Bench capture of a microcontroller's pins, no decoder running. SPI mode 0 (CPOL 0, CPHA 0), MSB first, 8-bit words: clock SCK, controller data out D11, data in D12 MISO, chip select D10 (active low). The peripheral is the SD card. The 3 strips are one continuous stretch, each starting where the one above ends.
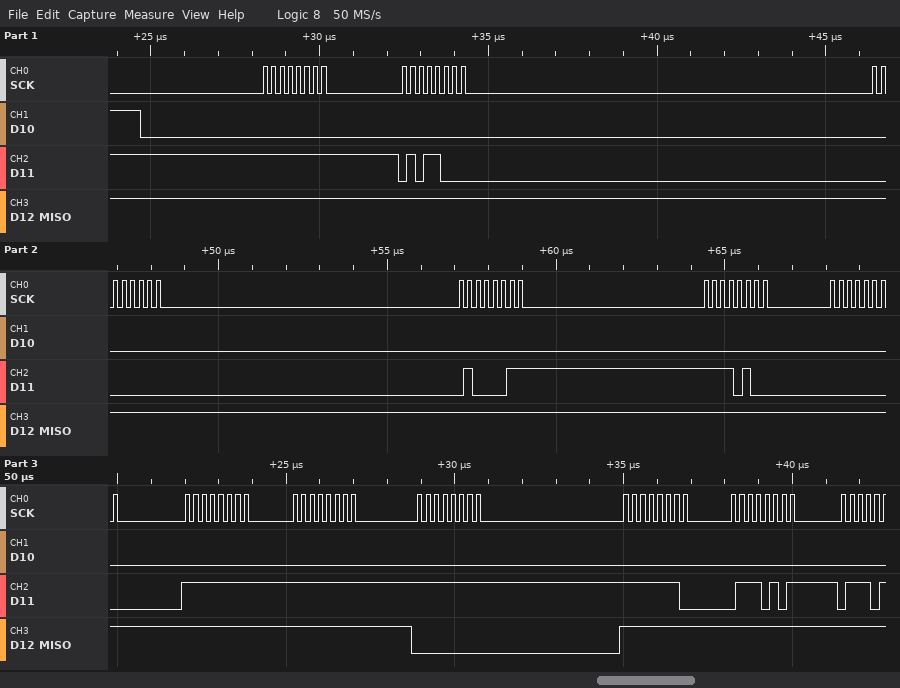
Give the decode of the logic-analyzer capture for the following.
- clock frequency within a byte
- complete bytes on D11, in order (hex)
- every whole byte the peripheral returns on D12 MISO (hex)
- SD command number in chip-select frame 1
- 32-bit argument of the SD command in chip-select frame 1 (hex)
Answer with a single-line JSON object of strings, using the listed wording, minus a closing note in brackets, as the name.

{"clock frequency within a byte": "4 MHz", "complete bytes on D11, in order": "FF 58 00 43 F4 00 FF FF FF FE 75", "every whole byte the peripheral returns on D12 MISO": "FF FF FF FF FF FF FF FF 00 FF FF", "SD command number in chip-select frame 1": "CMD24", "32-bit argument of the SD command in chip-select frame 1": "0x0043F400"}
